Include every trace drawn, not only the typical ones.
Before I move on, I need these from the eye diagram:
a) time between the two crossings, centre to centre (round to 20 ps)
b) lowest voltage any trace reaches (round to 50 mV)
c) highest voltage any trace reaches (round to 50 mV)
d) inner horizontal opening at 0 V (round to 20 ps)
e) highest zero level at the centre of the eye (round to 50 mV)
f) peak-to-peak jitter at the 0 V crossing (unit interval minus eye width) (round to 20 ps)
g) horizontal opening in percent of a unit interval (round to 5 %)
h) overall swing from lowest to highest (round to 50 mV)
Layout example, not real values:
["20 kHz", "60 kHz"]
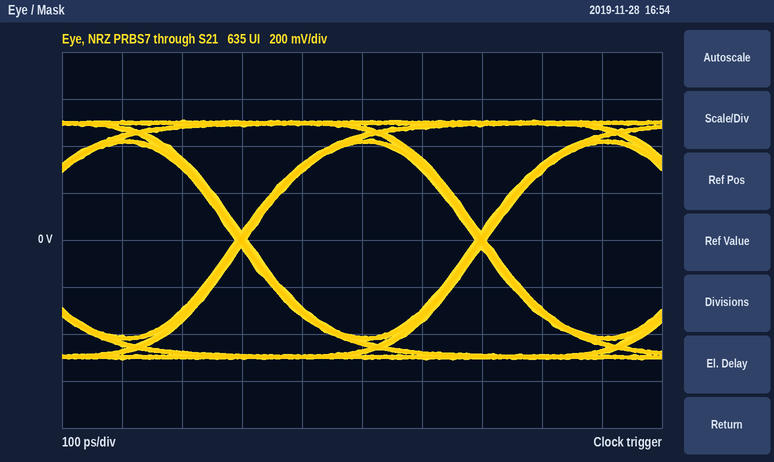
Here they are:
["400 ps", "-500 mV", "500 mV", "380 ps", "-400 mV", "20 ps", "95 %", "1.00 V"]
